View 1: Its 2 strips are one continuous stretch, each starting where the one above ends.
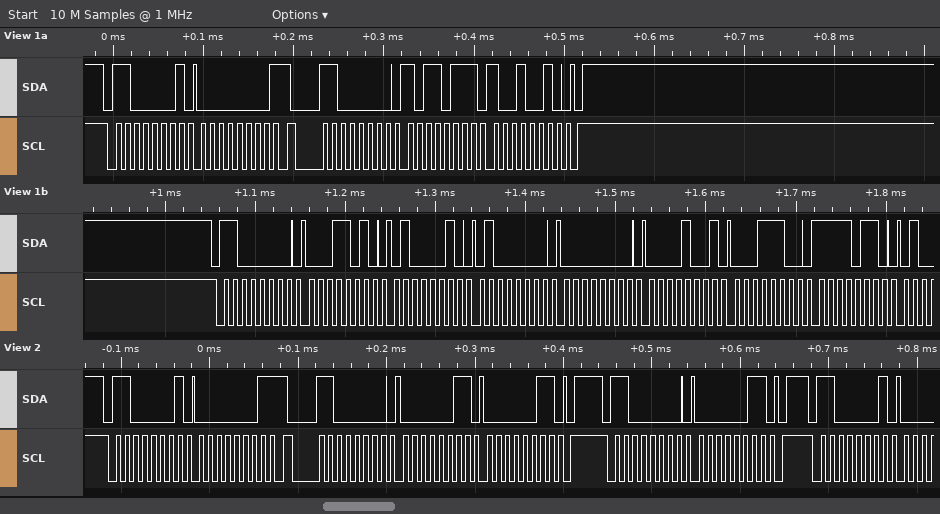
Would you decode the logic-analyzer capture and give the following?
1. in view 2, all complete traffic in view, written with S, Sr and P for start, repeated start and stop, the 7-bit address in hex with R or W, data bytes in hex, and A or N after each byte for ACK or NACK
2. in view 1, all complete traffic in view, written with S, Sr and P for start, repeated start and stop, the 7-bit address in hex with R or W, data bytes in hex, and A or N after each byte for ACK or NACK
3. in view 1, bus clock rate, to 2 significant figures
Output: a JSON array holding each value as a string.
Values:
["S 60R A 01 N Sr 60W A 03 A 03 A P S 60W A 03 A P S 60R A", "S 60R A 00 N Sr 60W A B7 A 92 A P S 60W A 1A A 42 A 40 A 00 A 09 A 1C A F6 A", "100 kHz"]
